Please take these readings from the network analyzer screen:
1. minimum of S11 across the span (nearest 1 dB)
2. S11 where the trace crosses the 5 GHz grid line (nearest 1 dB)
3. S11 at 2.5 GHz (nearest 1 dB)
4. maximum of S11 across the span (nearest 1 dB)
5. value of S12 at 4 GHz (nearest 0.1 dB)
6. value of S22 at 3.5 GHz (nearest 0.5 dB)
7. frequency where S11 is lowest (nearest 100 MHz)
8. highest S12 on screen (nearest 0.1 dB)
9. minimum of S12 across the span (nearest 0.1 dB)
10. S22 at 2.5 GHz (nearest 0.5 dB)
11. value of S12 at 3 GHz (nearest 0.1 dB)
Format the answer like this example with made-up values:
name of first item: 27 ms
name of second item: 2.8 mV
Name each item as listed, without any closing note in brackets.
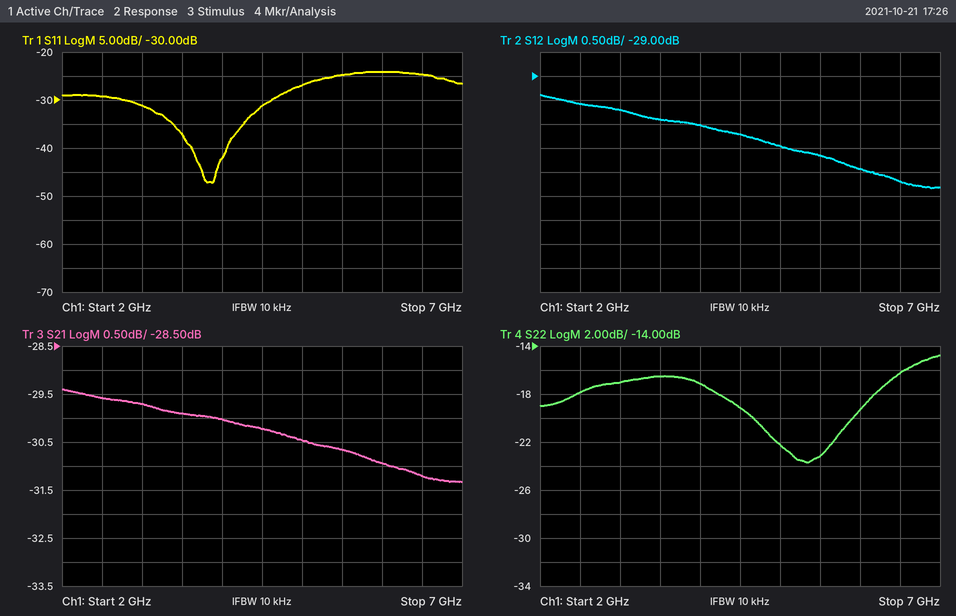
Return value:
minimum of S11 across the span: -47 dB
S11 where the trace crosses the 5 GHz grid line: -27 dB
S11 at 2.5 GHz: -29 dB
maximum of S11 across the span: -24 dB
value of S12 at 4 GHz: -30.0 dB
value of S22 at 3.5 GHz: -16.5 dB
frequency where S11 is lowest: 3.9 GHz
highest S12 on screen: -29.4 dB
minimum of S12 across the span: -31.3 dB
S22 at 2.5 GHz: -18.0 dB
value of S12 at 3 GHz: -29.7 dB
